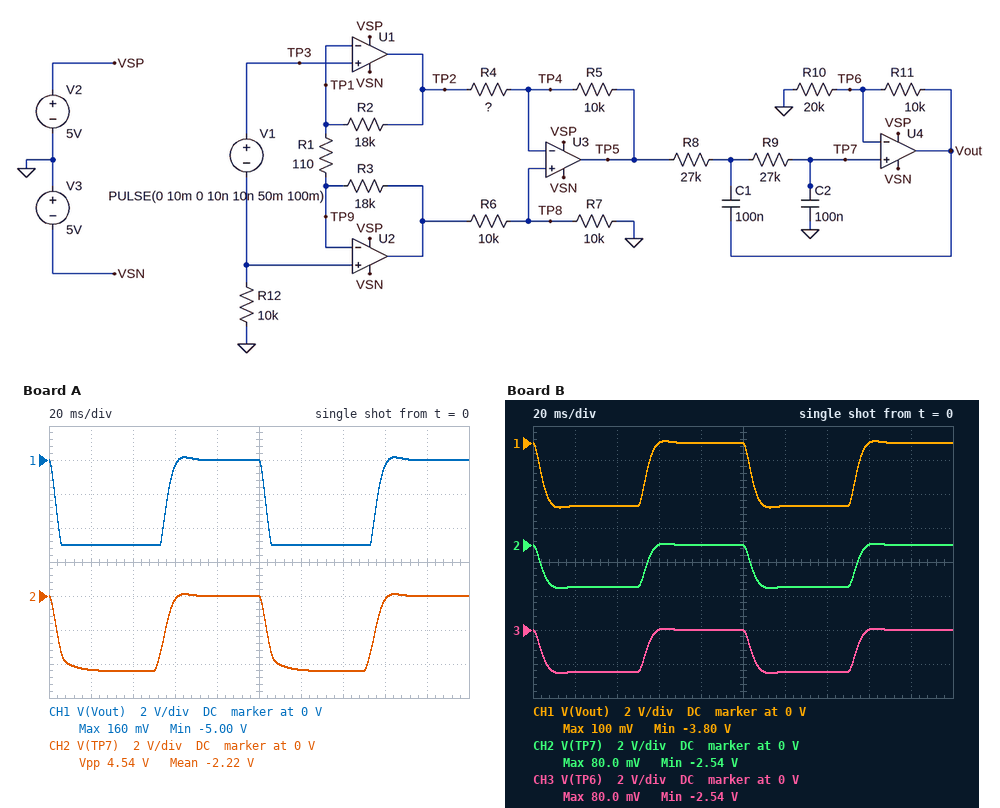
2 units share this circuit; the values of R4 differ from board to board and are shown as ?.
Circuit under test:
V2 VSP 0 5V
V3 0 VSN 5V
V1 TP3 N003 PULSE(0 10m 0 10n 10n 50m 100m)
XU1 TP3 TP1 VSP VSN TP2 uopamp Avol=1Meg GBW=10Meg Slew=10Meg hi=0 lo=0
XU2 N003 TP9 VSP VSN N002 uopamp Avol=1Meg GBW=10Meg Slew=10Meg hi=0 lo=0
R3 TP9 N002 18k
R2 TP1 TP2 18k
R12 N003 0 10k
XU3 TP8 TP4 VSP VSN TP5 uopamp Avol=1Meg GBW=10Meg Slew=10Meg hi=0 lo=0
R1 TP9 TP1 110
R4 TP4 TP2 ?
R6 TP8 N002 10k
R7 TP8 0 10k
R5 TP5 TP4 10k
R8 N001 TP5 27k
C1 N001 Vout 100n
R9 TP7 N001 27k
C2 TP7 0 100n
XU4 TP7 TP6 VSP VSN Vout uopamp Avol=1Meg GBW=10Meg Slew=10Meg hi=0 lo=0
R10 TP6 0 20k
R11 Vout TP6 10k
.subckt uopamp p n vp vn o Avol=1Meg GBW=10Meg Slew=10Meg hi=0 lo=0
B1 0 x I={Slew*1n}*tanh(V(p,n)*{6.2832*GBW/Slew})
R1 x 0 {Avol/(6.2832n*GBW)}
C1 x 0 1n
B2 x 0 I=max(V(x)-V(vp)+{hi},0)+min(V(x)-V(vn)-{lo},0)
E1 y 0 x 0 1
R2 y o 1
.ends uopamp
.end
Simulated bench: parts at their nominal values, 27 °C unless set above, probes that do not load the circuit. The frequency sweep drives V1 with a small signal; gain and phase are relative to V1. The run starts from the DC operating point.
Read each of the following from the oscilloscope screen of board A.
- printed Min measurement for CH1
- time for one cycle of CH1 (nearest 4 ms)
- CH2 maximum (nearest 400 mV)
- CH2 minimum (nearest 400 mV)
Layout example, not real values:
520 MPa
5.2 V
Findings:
-5.00 V
100 ms
0 V
-4.4 V
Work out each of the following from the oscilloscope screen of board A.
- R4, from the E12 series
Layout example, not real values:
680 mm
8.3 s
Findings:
6.8 kΩ
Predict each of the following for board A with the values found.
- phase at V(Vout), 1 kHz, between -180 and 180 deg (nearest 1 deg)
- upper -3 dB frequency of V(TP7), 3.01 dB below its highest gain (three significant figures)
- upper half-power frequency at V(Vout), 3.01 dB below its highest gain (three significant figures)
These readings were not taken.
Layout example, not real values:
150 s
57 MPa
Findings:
3 deg
55.4 Hz
55.4 Hz
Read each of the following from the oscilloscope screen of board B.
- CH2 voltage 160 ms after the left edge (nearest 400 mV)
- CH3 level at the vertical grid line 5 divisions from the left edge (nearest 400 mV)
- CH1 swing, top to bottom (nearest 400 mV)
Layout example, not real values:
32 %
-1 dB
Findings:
0 V
0 V
4.0 V
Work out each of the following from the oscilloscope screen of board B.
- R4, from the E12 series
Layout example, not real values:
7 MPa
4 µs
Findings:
15 kΩ
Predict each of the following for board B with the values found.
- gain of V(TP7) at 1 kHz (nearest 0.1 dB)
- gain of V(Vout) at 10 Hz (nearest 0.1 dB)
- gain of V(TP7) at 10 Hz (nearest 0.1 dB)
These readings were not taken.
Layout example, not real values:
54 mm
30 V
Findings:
-1.4 dB
51.3 dB
47.8 dB
